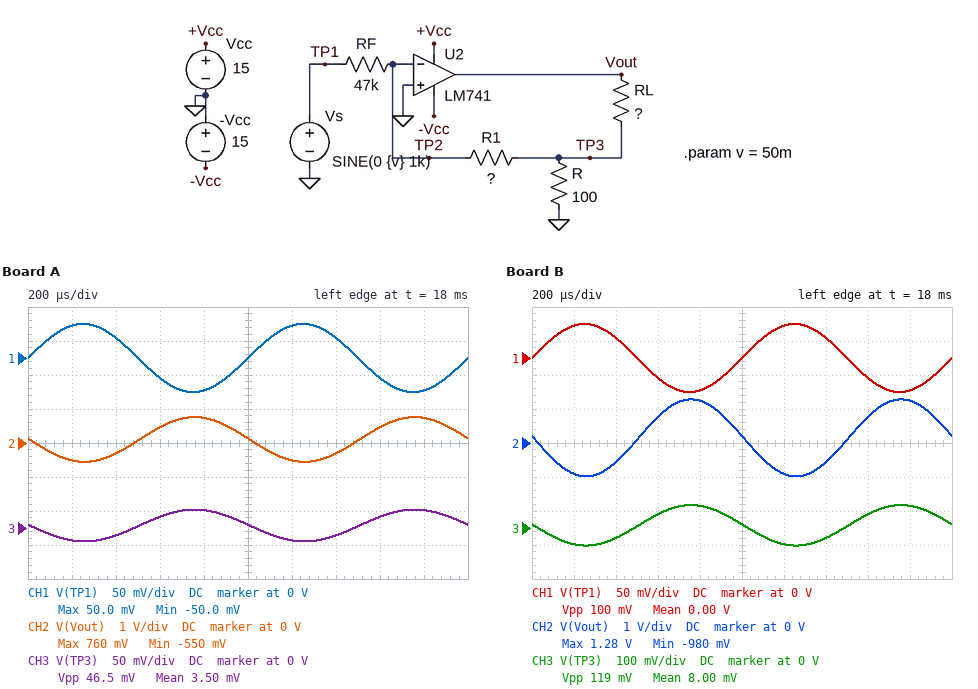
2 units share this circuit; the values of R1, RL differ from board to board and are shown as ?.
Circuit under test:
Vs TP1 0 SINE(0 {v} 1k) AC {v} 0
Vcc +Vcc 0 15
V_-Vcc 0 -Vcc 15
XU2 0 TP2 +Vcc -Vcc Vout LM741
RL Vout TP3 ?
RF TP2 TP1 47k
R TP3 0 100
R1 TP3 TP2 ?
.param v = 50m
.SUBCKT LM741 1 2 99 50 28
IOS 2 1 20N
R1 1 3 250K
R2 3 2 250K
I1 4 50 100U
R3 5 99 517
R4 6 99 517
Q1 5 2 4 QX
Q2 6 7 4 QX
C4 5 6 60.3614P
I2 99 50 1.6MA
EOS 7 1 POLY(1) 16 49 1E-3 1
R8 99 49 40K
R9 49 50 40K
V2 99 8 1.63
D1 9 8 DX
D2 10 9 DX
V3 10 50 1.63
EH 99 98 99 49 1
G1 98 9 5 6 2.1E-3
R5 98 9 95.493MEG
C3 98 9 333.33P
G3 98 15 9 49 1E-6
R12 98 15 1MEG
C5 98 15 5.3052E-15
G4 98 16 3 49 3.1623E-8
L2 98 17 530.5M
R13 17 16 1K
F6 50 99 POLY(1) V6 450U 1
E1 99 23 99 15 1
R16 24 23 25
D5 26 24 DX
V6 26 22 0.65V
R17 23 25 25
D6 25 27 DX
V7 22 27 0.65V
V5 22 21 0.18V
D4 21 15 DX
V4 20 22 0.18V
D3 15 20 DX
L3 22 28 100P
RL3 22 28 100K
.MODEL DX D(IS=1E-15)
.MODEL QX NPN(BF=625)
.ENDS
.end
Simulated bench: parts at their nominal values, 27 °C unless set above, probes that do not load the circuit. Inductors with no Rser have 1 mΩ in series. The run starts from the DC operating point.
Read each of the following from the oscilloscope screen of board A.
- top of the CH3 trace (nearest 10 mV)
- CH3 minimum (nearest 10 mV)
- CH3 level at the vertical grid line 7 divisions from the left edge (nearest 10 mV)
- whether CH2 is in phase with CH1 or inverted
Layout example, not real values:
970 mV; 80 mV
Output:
30 mV; -20 mV; -10 mV; inverted
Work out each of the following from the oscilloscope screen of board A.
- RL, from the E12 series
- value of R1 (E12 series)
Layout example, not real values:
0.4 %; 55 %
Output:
2.7 kΩ; 22 kΩ
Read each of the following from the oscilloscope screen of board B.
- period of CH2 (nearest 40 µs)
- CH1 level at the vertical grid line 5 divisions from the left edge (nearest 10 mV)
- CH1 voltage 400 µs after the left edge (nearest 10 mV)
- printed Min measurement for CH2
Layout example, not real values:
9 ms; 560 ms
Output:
1.00 ms; 0 V; 30 mV; -980 mV
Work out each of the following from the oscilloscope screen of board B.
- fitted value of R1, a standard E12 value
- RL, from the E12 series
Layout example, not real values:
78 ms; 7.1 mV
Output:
56 kΩ; 1.8 kΩ
